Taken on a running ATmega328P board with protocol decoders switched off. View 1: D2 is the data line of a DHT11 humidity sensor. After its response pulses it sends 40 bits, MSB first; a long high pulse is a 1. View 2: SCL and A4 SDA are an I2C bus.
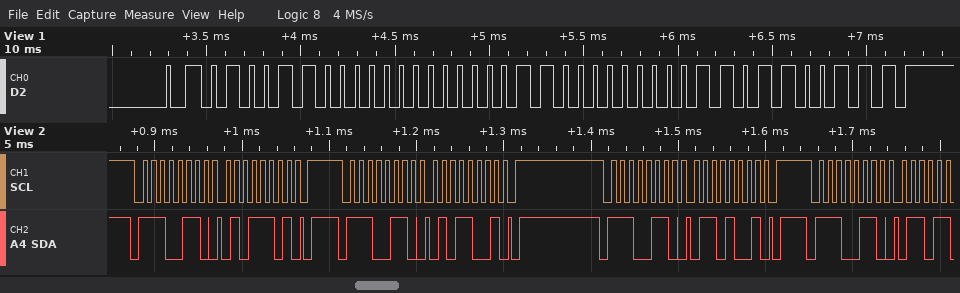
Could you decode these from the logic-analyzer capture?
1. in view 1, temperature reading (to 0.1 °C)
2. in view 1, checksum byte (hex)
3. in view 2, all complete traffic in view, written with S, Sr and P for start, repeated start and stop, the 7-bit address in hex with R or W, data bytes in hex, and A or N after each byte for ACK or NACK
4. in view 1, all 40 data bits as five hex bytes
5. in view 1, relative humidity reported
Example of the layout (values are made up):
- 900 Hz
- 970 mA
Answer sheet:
- 24.3 °C
- 0x67
- S 73W A 5D A P S 73W A 59 A P S 73W A 69 A P S 73W A
- 4C 00 18 03 67
- 76 %
